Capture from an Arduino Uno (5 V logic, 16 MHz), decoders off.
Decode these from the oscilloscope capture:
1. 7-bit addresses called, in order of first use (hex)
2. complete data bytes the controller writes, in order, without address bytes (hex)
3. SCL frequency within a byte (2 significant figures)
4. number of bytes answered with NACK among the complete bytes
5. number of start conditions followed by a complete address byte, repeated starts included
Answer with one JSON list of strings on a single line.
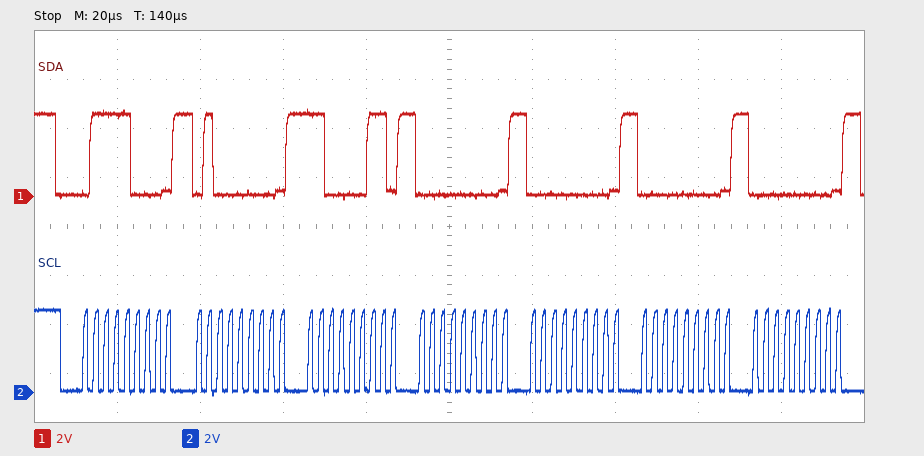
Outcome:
["0x3C", "40 C3 00 00 00 00", "400 kHz", "0", "1"]
